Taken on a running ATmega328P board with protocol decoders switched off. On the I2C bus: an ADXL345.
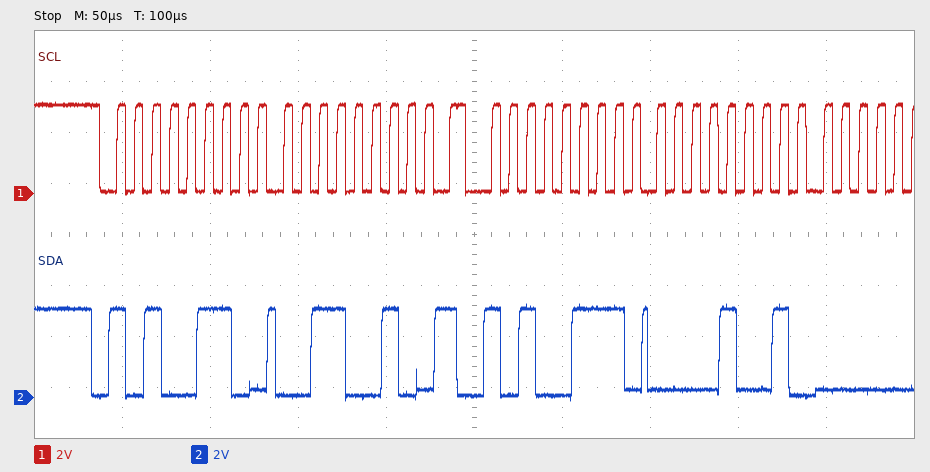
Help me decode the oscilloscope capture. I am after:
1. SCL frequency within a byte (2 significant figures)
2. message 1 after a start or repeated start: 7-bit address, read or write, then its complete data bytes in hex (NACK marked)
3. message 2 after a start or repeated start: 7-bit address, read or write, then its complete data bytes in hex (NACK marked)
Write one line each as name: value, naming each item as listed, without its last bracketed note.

SCL frequency within a byte: 100 kHz
message 1 after a start or repeated start: 7-bit address, read or write, then its complete data bytes in hex: 0x53 write: 32
message 2 after a start or repeated start: 7-bit address, read or write, then its complete data bytes in hex: 0x53 read: 09
